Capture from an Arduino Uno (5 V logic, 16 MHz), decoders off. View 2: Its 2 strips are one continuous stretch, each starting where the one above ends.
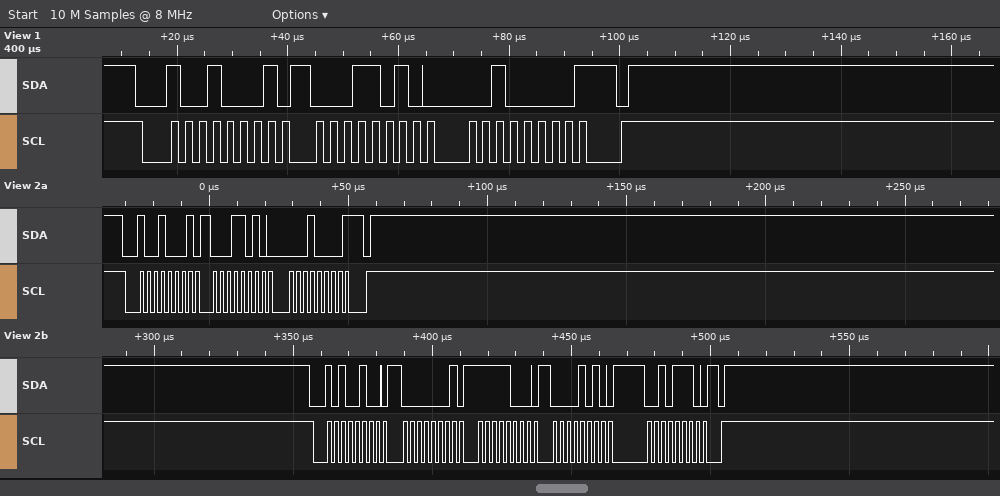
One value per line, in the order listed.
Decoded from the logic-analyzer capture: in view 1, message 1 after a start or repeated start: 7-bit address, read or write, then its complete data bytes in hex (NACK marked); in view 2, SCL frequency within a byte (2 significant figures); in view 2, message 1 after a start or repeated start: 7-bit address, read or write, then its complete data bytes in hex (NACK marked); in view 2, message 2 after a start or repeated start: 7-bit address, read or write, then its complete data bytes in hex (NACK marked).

0x48 read: 1A 20 NACK
400 kHz
0x48 read: 1A 10 NACK
0x52 write: 01 F8 0A 2E
